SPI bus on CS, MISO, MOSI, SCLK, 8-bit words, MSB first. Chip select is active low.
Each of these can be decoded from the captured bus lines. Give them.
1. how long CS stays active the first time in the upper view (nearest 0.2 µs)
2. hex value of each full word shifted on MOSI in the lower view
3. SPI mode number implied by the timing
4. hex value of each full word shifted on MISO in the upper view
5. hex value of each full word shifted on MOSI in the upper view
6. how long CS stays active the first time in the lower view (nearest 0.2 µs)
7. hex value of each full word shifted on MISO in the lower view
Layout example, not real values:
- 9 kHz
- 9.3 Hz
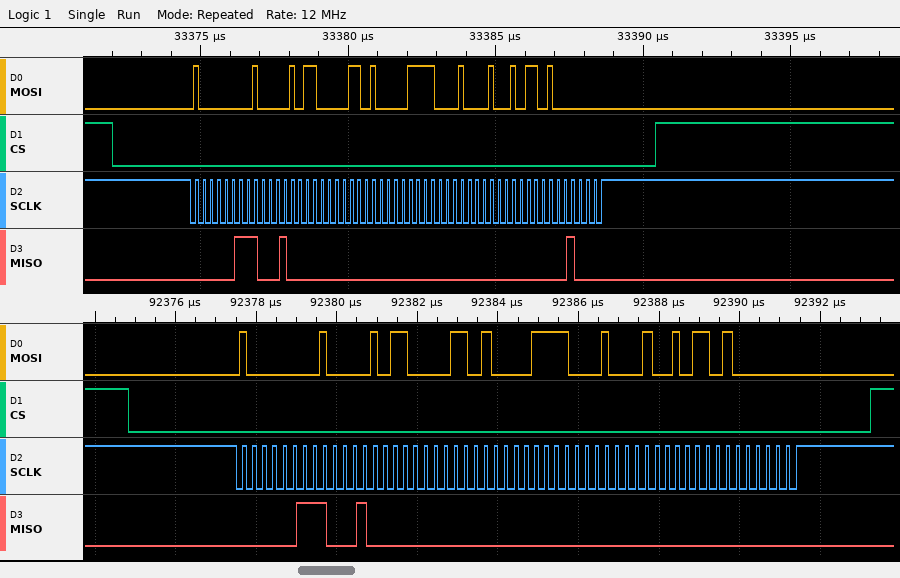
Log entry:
- 18.4 µs
- 80, 85, 86, 87, 88, 96, 80
- 3
- 03, 88, 00, 00, 00, 00, 10
- 80, 85, 86, 87, 88, 96, 80
- 18.4 µs
- 03, 88, 00, 00, 00, 00, 00
